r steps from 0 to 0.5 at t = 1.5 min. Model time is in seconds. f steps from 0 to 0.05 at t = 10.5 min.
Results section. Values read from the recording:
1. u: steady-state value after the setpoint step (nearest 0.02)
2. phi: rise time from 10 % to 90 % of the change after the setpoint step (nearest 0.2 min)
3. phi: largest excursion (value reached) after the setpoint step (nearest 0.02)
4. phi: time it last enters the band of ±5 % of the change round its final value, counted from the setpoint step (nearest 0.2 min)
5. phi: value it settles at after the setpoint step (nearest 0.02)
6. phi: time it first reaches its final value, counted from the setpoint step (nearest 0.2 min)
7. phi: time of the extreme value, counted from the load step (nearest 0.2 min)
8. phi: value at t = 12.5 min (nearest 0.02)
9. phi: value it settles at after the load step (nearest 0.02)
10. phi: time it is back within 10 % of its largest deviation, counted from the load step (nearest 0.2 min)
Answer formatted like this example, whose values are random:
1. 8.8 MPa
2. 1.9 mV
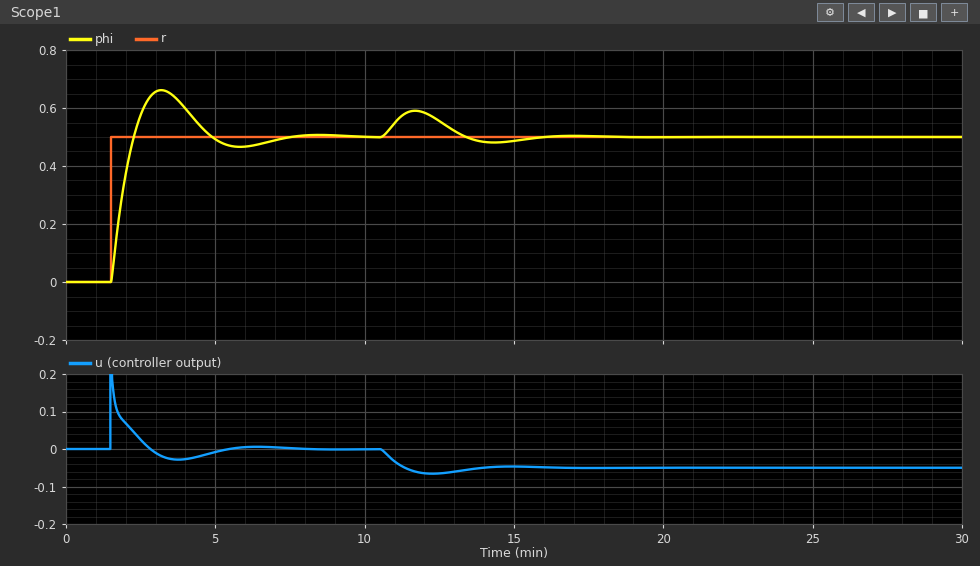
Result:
1. 0.00
2. 0.6 min
3. 0.66
4. 5.0 min
5. 0.50
6. 0.8 min
7. 1.2 min
8. 0.56
9. 0.50
10. 4.8 min
